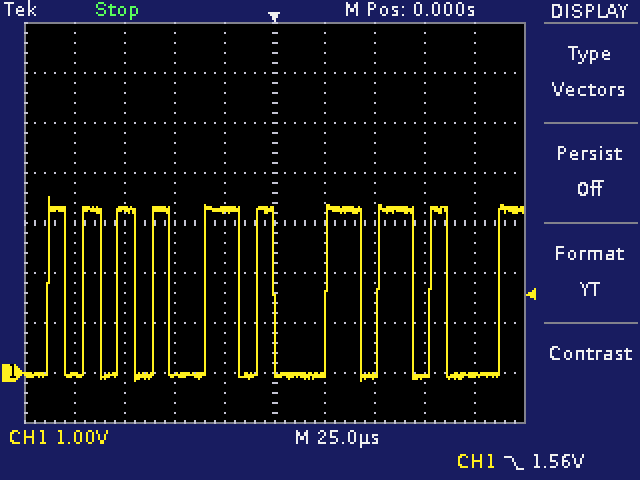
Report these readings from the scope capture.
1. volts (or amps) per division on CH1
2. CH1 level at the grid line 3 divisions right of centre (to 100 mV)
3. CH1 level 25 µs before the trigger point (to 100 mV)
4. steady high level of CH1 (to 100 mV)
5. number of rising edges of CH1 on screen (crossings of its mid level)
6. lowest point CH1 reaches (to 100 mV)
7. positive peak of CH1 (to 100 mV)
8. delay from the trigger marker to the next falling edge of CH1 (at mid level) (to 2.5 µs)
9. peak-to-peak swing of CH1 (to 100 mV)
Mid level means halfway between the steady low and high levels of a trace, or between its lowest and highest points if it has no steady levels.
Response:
1 V
-100 mV
3.3 V
3.3 V
10
-200 mV
3.5 V
42.5 µs
3.7 V
